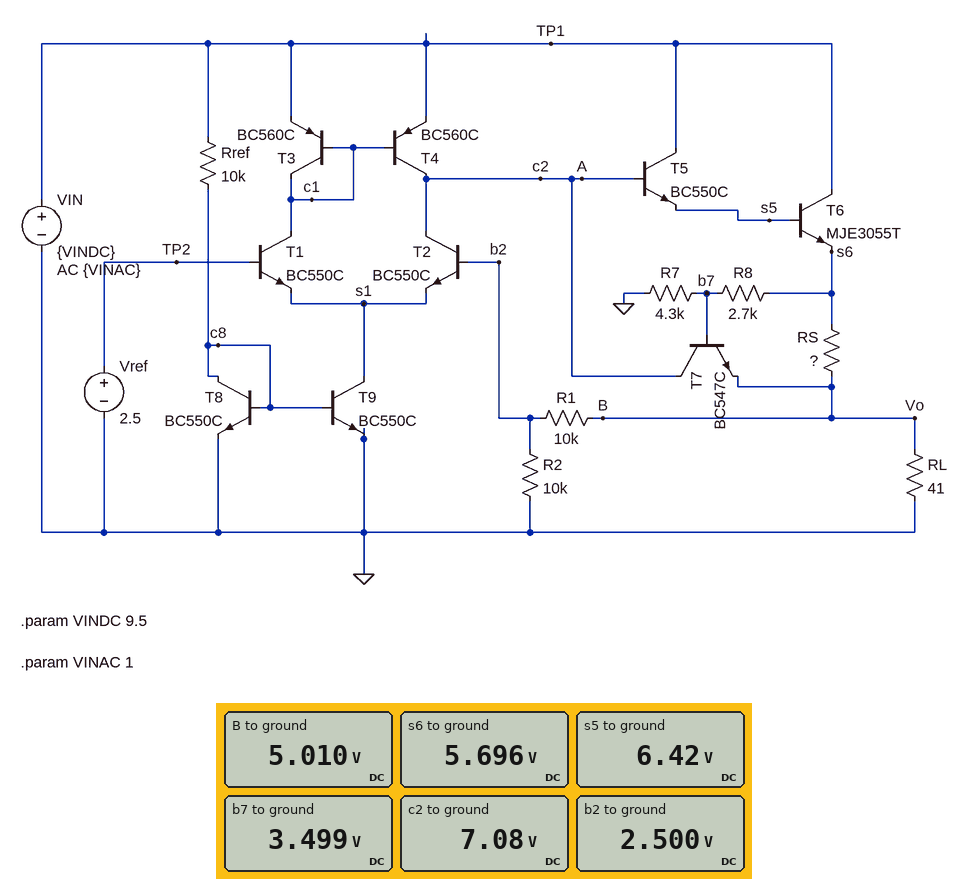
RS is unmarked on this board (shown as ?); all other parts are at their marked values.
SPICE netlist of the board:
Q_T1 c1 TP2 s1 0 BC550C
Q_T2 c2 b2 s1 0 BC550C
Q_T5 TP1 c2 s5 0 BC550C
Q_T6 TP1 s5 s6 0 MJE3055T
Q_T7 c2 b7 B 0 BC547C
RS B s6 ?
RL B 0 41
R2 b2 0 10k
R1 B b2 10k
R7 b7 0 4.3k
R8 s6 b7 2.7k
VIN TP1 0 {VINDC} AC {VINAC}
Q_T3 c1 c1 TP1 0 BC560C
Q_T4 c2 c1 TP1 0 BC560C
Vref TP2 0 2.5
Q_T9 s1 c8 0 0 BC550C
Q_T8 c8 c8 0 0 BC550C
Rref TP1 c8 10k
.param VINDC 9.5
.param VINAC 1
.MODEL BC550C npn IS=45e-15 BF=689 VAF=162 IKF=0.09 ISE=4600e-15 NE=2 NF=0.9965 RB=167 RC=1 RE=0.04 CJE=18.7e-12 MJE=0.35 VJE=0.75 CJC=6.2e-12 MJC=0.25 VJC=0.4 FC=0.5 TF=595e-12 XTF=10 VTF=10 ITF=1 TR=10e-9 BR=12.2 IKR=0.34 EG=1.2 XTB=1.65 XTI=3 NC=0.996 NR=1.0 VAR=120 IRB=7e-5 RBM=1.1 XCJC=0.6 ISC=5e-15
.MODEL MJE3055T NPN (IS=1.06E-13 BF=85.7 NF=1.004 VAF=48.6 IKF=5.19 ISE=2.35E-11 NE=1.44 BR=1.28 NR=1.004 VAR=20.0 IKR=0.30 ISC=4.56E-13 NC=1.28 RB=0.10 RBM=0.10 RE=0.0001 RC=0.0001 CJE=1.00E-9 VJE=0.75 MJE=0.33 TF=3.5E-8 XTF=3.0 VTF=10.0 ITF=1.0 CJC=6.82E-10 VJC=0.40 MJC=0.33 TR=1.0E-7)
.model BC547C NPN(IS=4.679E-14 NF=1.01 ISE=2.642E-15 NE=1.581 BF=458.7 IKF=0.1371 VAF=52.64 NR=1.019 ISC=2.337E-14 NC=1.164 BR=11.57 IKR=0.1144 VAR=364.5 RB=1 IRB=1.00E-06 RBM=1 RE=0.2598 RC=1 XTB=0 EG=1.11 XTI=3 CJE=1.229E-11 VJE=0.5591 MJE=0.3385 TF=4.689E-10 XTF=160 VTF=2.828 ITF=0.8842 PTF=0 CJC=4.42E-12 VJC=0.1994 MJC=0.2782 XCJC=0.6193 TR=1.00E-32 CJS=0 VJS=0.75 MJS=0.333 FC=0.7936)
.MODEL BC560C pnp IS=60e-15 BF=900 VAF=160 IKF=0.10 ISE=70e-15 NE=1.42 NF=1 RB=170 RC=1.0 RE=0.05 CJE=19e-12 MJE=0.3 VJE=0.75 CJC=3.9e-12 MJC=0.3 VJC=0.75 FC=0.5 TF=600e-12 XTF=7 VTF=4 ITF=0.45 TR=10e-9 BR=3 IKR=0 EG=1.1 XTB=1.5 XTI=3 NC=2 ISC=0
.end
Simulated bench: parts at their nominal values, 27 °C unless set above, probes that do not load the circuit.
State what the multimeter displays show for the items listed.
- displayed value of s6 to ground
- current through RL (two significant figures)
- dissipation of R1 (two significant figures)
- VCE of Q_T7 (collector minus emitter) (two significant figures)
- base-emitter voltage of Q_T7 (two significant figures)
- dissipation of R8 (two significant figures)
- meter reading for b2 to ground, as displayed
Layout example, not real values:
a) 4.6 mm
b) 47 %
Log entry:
a) 5.696 V
b) 120 mA
c) 630 µW
d) 2.1 V
e) -1.5 V
f) 1.8 mW
g) 2.500 V
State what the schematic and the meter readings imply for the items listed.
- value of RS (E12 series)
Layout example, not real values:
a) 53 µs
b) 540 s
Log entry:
a) 5.6 Ω
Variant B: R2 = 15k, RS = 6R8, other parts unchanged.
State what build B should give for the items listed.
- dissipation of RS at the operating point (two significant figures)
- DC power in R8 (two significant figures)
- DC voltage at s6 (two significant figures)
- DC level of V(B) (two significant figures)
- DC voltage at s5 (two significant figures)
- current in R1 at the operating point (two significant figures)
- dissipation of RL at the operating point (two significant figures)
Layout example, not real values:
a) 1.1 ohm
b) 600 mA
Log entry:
a) 71 mW
b) 1.3 mW
c) 4.9 V
d) 4.2 V
e) 5.6 V
f) 170 µA
g) 430 mW
